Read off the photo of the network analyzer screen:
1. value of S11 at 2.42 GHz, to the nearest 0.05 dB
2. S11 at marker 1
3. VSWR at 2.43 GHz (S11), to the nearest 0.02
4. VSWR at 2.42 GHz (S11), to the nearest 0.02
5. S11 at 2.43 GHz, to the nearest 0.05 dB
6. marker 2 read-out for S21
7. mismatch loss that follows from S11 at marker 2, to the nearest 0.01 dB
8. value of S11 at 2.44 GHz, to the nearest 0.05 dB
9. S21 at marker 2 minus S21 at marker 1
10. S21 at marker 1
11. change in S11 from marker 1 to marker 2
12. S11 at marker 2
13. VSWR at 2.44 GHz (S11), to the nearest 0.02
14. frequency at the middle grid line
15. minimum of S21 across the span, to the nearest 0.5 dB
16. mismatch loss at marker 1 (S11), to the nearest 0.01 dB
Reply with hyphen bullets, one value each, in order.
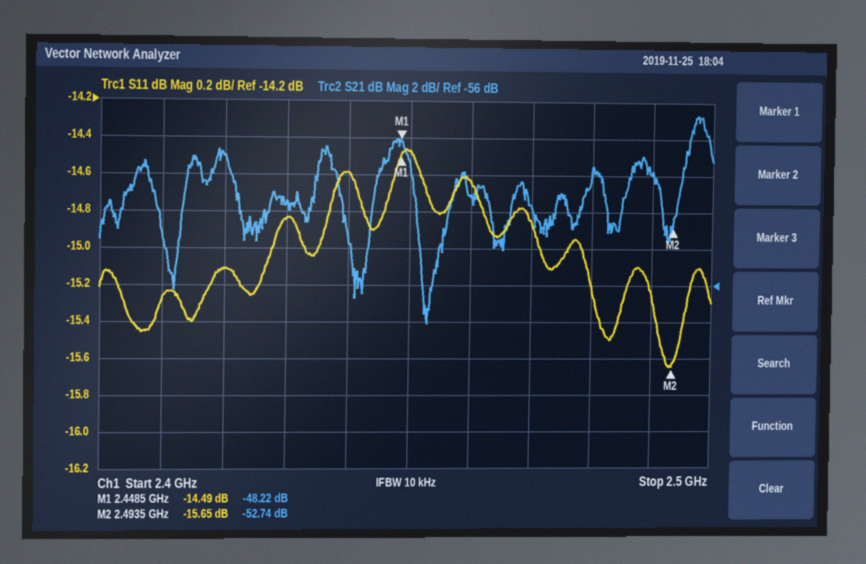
- -15.10 dB
- -14.49 dB
- 1.44
- 1.42
- -14.85 dB
- -52.74 dB
- 0.12 dB
- -14.60 dB
- -4.52 dB
- -48.22 dB
- -1.16 dB
- -15.65 dB
- 1.46
- 2.45 GHz
- -58.0 dB
- 0.16 dB
